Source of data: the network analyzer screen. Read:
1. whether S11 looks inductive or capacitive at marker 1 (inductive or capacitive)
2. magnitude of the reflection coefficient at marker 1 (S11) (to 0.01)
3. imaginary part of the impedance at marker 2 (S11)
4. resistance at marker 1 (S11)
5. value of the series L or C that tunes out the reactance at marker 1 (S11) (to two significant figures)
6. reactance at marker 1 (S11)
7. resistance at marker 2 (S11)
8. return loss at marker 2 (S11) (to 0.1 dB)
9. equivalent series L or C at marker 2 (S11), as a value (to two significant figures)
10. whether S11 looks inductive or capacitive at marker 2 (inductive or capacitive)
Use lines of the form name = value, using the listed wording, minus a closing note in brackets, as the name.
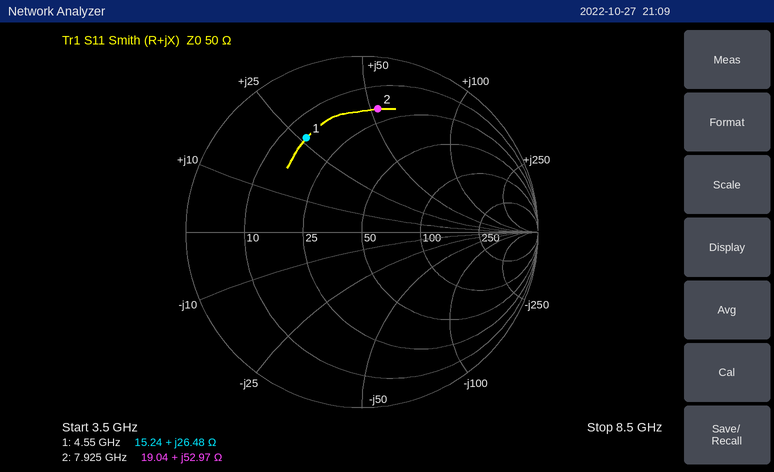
whether S11 looks inductive or capacitive at marker 1 = inductive
magnitude of the reflection coefficient at marker 1 (S11) = 0.62
imaginary part of the impedance at marker 2 = +52.97 Ω
resistance at marker 1 = 15.24 Ω
value of the series L or C that tunes out the reactance at marker 1 (S11) = 1.3 pF
reactance at marker 1 = +26.48 Ω
resistance at marker 2 = 19.04 Ω
return loss at marker 2 (S11) = 3.0 dB
equivalent series L or C at marker 2 (S11), as a value = 1.1 nH
whether S11 looks inductive or capacitive at marker 2 = inductive
